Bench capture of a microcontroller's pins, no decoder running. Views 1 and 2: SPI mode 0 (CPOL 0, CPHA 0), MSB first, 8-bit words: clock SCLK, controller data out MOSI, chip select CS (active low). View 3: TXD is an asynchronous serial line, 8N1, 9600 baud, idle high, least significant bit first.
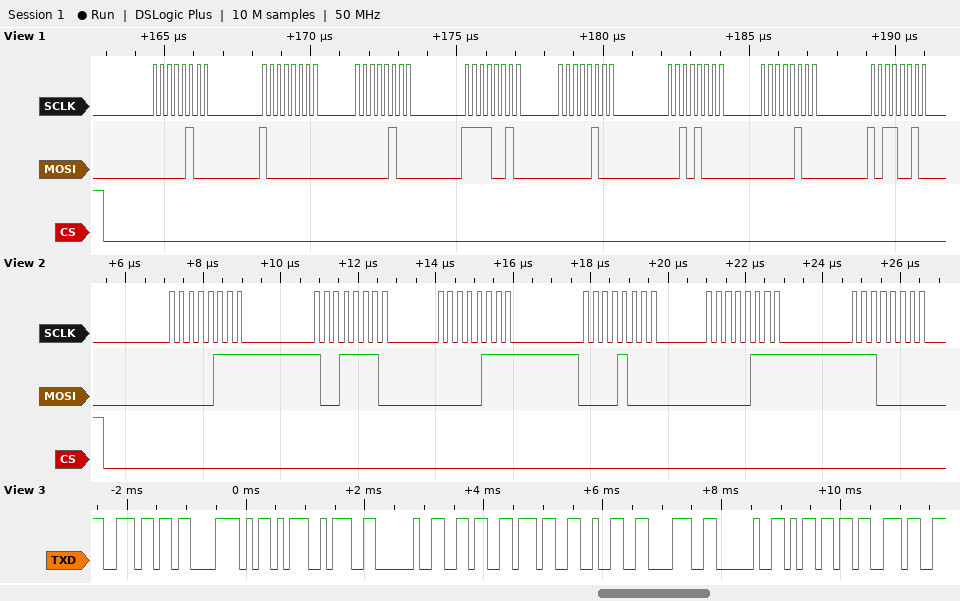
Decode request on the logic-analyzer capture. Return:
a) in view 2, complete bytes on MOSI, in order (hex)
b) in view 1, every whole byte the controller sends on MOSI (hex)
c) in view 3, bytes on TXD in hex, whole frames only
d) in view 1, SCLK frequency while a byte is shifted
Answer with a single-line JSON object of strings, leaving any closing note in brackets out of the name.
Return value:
{"in view 2, complete bytes on MOSI, in order": "07 9E 07 08 07 E0", "in view 1, every whole byte the controller sends on MOSI": "0x04 0x80 0x04 0xF2 0x04 0x28 0x04 0xB2", "in view 3, bytes on TXD in hex, whole frames only": "6E C3 AD 3A 20 36 37 32 38 20 6D 73", "in view 1, SCLK frequency while a byte is shifted": "4 MHz"}
